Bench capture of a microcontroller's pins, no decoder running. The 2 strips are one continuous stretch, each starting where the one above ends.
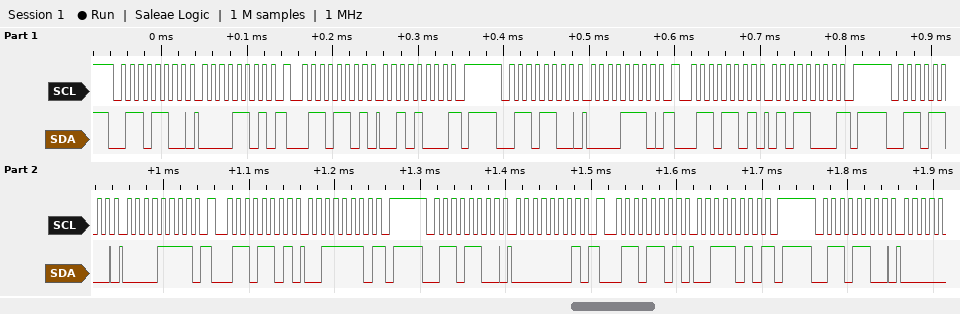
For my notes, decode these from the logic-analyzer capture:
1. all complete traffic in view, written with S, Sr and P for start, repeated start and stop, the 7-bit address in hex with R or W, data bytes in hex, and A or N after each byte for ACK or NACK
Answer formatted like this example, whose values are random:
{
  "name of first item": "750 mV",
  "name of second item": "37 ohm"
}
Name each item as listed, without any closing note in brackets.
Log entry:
{
  "all complete traffic in view, written with S, Sr and P for start, repeated start and stop, the 7-bit address in hex with R or W, data bytes in hex, and A or N after each byte for ACK or NACK": "S 36W A 0D A Sr 36R A 28 N P S 36W A 0E A Sr 36R A 58 N P S 36W A 0F A Sr 36R A 3E N P S 36W A 01 A Sr 36R A 3A N P S 36W A"
}
